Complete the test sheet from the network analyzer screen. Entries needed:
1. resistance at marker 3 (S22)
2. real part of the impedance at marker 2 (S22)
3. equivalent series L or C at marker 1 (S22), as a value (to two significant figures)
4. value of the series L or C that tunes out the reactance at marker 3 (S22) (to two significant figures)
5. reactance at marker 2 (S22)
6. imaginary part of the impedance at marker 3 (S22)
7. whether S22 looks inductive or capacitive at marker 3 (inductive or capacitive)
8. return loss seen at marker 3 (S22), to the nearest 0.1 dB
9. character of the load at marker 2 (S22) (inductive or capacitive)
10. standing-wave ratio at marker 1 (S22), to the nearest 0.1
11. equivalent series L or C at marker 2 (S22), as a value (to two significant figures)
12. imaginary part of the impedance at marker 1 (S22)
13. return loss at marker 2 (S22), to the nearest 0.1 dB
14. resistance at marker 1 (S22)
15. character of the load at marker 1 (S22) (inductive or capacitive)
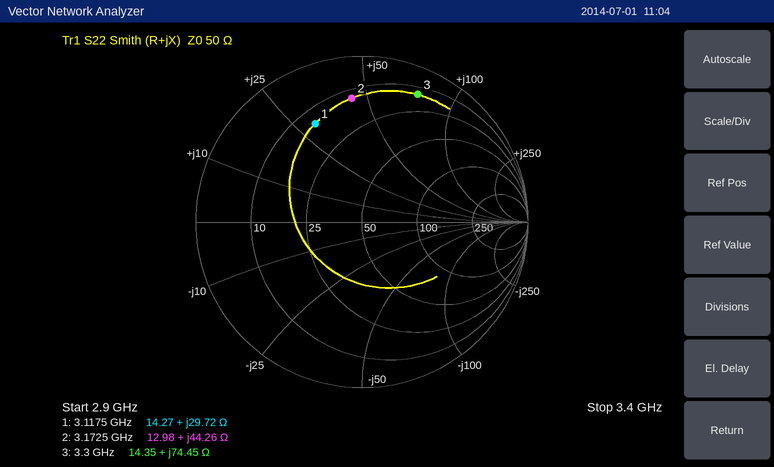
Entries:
14.35 Ω
12.98 Ω
1.5 nH
650 fF
+44.26 Ω
+74.45 Ω
inductive
1.5 dB
inductive
4.8
2.2 nH
+29.72 Ω
2.5 dB
14.27 Ω
inductive
